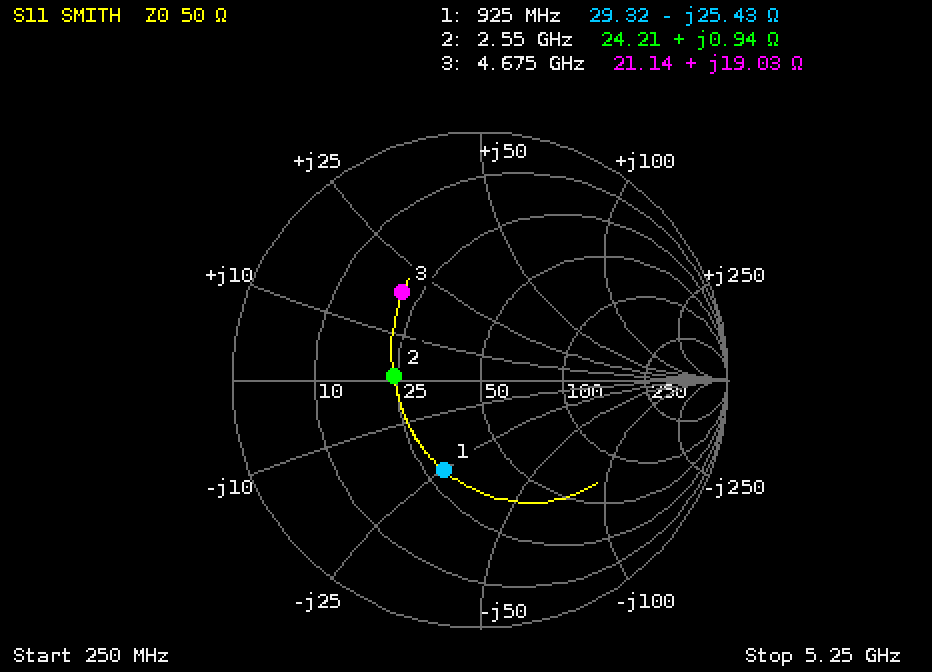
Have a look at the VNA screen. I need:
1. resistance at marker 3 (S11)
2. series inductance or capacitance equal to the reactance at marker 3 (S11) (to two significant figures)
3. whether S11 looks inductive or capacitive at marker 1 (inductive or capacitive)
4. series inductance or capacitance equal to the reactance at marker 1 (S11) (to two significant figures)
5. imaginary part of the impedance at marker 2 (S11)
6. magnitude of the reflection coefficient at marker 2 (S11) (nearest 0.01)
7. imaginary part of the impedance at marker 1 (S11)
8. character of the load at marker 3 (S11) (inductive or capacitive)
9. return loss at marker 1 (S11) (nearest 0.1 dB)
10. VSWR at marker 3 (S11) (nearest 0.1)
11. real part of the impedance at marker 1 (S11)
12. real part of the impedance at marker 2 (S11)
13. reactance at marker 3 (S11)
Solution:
21.14 Ω
650 pH
capacitive
6.8 pF
+0.94 Ω
0.35
-25.43 Ω
inductive
8.1 dB
2.8
29.32 Ω
24.21 Ω
+19.03 Ω
